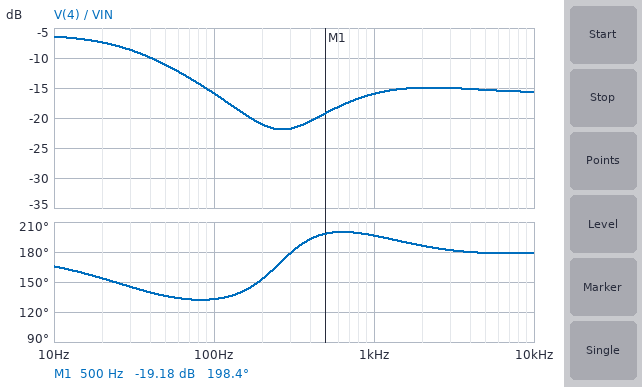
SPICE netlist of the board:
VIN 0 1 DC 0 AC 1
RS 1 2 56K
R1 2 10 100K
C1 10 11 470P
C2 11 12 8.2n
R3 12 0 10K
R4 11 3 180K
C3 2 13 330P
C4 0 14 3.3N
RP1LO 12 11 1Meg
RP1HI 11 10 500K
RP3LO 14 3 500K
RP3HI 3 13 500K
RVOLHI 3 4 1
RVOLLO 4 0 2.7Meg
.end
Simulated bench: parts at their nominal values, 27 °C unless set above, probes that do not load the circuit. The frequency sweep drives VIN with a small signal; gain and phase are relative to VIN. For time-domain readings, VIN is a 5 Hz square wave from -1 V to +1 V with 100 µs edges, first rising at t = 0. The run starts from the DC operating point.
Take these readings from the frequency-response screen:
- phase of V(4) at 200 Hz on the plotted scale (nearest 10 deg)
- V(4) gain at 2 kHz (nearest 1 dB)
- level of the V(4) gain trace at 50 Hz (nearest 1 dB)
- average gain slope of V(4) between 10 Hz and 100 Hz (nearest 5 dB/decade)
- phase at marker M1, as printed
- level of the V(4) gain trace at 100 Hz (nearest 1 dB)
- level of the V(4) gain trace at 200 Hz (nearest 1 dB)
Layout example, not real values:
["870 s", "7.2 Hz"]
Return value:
["150 deg", "-15 dB", "-11 dB", "-10 dB/decade", "198.4 deg", "-16 dB", "-21 dB"]
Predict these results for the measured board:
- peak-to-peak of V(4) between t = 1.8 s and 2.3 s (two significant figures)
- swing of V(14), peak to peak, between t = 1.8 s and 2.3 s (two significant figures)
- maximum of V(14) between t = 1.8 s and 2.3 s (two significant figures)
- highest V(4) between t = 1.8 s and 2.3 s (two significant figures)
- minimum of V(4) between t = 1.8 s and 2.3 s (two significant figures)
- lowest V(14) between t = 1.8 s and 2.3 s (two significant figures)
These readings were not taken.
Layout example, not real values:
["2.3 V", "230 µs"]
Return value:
["1.0 V", "1.0 V", "500 mV", "500 mV", "-500 mV", "-500 mV"]
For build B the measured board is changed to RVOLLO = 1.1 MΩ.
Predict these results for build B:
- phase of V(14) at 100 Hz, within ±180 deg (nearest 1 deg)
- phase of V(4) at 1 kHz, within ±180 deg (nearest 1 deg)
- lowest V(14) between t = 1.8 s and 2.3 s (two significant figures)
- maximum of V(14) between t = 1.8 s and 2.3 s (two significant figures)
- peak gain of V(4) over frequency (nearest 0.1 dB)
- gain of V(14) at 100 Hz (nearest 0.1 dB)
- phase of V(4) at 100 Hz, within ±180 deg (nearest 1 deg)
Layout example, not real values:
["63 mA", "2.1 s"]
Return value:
["90 deg", "-163 deg", "-400 mV", "400 mV", "-8.0 dB", "-19.8 dB", "136 deg"]
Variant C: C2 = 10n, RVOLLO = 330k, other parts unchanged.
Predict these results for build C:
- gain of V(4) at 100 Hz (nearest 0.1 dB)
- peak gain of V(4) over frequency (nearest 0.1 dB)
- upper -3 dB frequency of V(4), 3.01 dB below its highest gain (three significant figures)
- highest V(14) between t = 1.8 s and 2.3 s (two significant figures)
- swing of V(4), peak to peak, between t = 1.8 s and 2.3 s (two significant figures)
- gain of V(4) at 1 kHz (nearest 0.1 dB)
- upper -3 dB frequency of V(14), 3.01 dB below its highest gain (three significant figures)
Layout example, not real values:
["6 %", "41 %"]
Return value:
["-20.4 dB", "-13.1 dB", "49.5 Hz", "220 mV", "440 mV", "-18.4 dB", "41.2 Hz"]
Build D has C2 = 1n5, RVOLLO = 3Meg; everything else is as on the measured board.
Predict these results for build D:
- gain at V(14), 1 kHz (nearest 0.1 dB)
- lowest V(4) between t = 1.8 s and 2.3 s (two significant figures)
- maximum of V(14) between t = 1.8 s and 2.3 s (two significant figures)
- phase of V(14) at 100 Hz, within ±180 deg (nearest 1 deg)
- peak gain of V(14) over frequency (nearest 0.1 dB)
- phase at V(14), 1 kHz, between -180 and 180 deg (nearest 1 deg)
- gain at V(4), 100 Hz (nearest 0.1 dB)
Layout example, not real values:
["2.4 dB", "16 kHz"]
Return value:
["-32.3 dB", "-510 mV", "510 mV", "114 deg", "-5.9 dB", "91 deg", "-10.5 dB"]
